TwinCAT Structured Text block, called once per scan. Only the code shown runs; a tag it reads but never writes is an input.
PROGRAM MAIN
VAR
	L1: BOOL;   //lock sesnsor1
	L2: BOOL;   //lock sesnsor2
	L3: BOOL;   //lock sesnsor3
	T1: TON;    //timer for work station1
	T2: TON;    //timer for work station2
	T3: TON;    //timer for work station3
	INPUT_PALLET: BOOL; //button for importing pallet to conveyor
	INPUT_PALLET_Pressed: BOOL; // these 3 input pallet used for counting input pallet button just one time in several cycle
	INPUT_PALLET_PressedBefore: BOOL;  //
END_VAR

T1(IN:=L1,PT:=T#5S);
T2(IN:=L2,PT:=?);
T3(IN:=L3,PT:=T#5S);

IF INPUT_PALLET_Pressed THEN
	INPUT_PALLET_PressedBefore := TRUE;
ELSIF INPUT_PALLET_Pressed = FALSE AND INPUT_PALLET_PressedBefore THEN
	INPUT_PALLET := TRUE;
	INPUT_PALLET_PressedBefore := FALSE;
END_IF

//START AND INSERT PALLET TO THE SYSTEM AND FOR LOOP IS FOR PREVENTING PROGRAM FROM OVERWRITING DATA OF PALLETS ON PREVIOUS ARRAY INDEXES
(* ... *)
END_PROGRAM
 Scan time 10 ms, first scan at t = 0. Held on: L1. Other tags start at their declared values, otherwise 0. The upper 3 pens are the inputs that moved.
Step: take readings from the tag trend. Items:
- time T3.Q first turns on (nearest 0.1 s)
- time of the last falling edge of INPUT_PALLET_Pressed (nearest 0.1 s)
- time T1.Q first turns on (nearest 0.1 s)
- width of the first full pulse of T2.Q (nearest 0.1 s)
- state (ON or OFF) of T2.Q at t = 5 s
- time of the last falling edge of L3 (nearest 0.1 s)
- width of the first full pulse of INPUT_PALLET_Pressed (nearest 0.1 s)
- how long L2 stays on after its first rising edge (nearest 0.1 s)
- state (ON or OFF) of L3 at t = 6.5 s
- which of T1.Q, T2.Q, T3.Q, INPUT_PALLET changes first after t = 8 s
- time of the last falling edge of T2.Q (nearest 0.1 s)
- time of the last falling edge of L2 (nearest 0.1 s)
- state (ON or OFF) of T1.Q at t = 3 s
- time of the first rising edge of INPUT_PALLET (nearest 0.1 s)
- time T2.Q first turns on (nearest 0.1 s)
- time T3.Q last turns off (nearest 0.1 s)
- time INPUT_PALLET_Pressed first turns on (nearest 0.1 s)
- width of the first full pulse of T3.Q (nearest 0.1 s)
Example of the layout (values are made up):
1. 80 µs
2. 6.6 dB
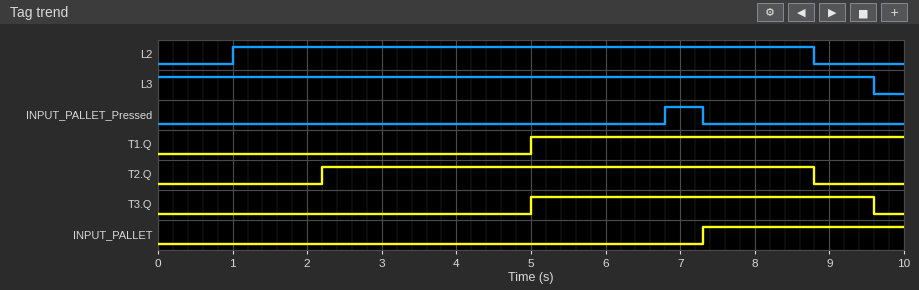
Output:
1. 5.0 s
2. 7.3 s
3. 5.0 s
4. 6.6 s
5. ON
6. 9.6 s
7. 0.5 s
8. 7.8 s
9. ON
10. T2.Q
11. 8.8 s
12. 8.8 s
13. OFF
14. 7.3 s
15. 2.2 s
16. 9.6 s
17. 6.8 s
18. 4.6 s
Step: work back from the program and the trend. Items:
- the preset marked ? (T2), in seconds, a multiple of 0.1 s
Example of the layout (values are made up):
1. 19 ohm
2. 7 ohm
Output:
1. 1.2 s
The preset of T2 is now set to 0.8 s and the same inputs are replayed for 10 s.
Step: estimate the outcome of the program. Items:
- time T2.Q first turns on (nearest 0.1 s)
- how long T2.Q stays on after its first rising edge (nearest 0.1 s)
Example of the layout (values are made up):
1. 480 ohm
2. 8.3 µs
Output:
1. 1.8 s
2. 7.0 s
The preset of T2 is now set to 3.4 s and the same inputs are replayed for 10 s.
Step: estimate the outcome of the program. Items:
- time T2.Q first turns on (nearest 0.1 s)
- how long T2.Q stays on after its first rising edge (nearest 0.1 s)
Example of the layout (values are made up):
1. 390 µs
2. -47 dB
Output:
1. 4.4 s
2. 4.4 s
